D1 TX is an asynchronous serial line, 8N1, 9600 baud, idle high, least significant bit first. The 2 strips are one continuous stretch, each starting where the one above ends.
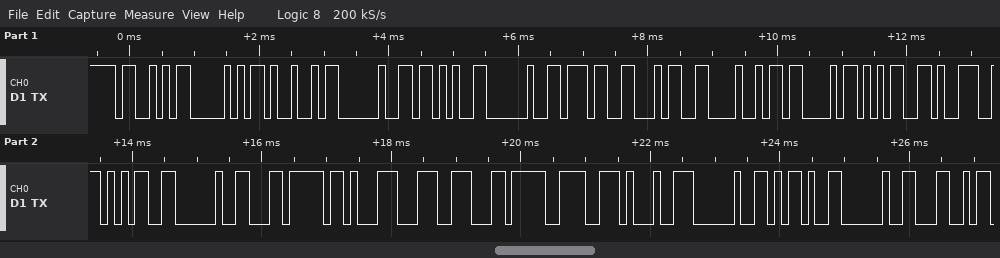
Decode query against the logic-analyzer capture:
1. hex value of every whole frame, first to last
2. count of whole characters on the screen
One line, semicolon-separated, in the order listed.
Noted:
53 50 49 20 2B 20 37 34 48 43 35 39 35 20 EC 8B 9C EC 9E 91 20 2D 20 4C; 24
